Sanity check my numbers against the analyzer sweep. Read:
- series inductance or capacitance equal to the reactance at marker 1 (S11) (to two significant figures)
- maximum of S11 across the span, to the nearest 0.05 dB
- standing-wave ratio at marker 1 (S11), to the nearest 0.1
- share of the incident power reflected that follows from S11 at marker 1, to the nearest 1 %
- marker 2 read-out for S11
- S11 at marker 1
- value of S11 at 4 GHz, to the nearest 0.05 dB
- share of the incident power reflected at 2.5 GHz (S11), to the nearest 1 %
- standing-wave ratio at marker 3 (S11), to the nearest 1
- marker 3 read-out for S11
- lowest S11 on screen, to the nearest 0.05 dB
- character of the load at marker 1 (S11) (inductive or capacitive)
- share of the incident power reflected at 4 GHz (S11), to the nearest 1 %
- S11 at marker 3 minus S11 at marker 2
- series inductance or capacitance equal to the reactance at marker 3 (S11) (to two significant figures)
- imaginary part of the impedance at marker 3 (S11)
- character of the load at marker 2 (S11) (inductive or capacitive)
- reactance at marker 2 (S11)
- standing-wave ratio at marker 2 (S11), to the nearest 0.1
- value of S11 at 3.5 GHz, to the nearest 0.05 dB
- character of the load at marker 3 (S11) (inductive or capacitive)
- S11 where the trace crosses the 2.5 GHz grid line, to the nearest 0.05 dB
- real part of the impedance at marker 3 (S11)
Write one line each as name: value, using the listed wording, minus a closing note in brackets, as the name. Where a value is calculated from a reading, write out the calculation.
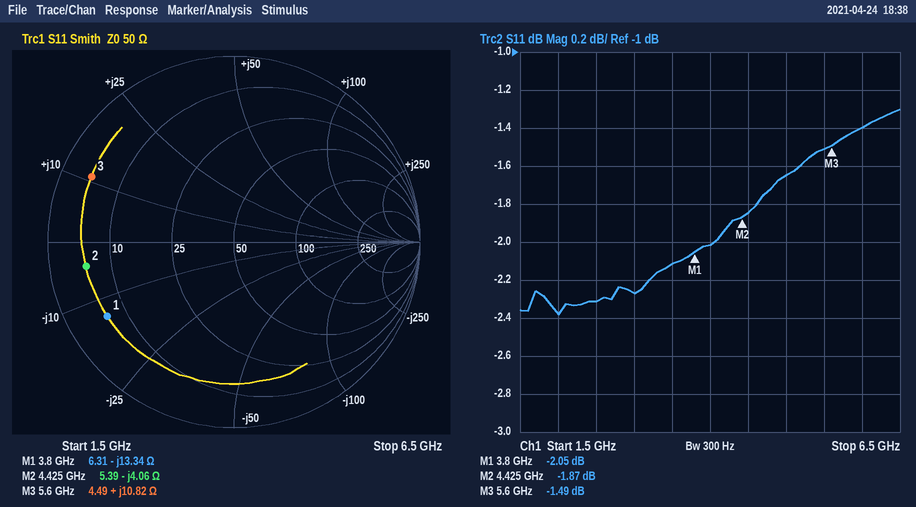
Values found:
series inductance or capacitance equal to the reactance at marker 1 (S11): C = 1/(2π × 3.8 GHz × 13.34 Ω) ≈ 3.1 pF
maximum of S11 across the span, to the nearest 0.05 dB: -1.30 dB
standing-wave ratio at marker 1 (S11), to the nearest 0.1: 8.5
share of the incident power reflected that follows from S11 at marker 1, to the nearest 1 %: 10^(-2.05/10) ≈ 62 %
marker 2 read-out for S11: -1.87 dB
S11 at marker 1: -2.05 dB
value of S11 at 4 GHz, to the nearest 0.05 dB: -2.00 dB
share of the incident power reflected at 2.5 GHz (S11), to the nearest 1 %: 10^(-2.3/10) ≈ 59 %
standing-wave ratio at marker 3 (S11), to the nearest 1: 12
marker 3 read-out for S11: -1.49 dB
lowest S11 on screen, to the nearest 0.05 dB: -2.40 dB
character of the load at marker 1 (S11): capacitive
share of the incident power reflected at 4 GHz (S11), to the nearest 1 %: 10^(-2/10) ≈ 63 %
S11 at marker 3 minus S11 at marker 2: -1.49 − (-1.87) = 0.38 dB
series inductance or capacitance equal to the reactance at marker 3 (S11): L = 10.82 Ω/(2π × 5.6 GHz) ≈ 308 pH, so 310 pH to two significant figures
imaginary part of the impedance at marker 3: +10.82 Ω
character of the load at marker 2 (S11): capacitive
reactance at marker 2: -4.06 Ω
standing-wave ratio at marker 2 (S11), to the nearest 0.1: 9.3
value of S11 at 3.5 GHz, to the nearest 0.05 dB: -2.10 dB
character of the load at marker 3 (S11): inductive
S11 where the trace crosses the 2.5 GHz grid line, to the nearest 0.05 dB: -2.30 dB
real part of the impedance at marker 3: 4.49 Ω
